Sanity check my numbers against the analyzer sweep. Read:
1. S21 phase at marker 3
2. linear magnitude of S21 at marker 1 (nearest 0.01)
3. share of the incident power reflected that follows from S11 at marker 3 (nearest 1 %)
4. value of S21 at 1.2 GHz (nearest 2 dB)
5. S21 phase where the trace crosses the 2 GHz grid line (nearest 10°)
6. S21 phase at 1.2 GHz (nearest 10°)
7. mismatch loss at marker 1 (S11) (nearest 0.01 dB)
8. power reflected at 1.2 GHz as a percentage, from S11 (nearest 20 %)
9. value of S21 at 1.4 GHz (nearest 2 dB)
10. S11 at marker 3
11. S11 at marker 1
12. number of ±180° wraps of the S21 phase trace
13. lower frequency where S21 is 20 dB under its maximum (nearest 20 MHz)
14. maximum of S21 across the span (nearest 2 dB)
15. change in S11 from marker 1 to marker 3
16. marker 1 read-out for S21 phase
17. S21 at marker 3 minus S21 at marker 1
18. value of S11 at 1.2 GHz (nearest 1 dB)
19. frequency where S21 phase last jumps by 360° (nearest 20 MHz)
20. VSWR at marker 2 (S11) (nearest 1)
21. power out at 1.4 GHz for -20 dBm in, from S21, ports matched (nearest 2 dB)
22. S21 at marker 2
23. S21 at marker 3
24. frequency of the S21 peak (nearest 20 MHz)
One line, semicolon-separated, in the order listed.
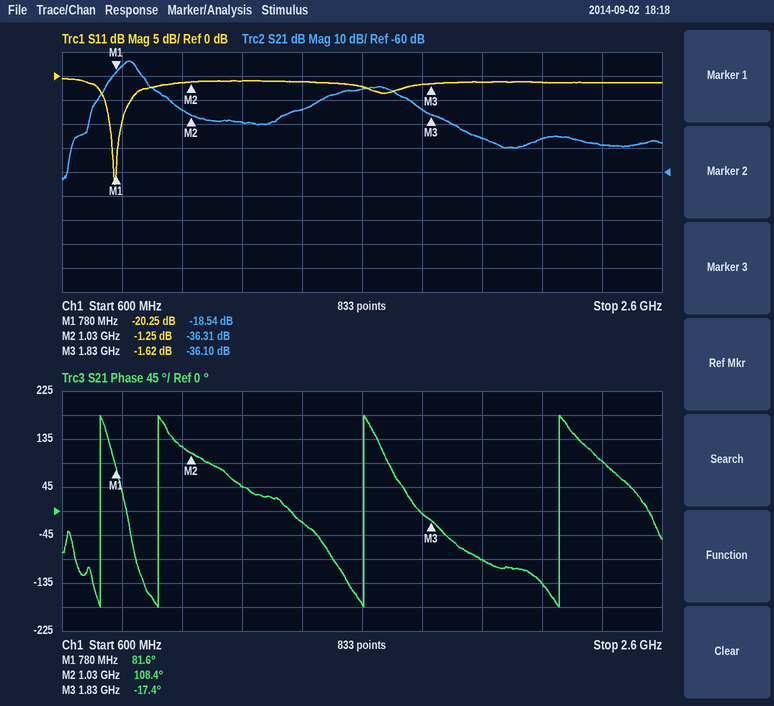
-17.4°; 0.12; 69 %; -40 dB; -90°; 50°; 0.04 dB; 80 %; -34 dB; -1.62 dB; -20.25 dB; 4; 700 MHz; -14 dB; 18.63 dB; 81.6°; -17.56 dB; -1 dB; 2.26 GHz; 14; -54 dBm; -36.31 dB; -36.10 dB; 820 MHz
